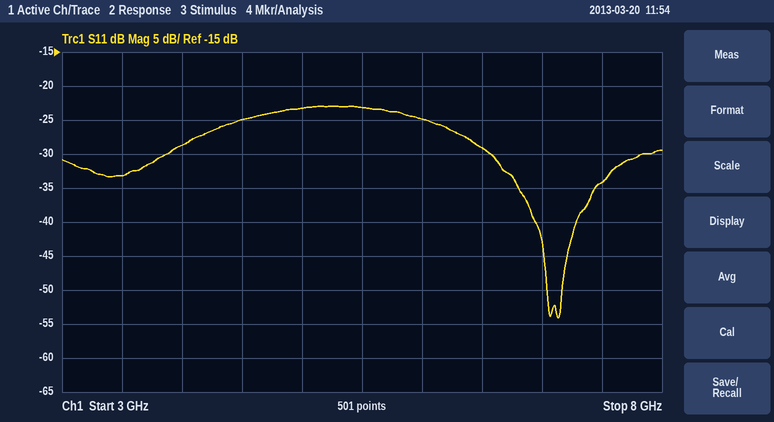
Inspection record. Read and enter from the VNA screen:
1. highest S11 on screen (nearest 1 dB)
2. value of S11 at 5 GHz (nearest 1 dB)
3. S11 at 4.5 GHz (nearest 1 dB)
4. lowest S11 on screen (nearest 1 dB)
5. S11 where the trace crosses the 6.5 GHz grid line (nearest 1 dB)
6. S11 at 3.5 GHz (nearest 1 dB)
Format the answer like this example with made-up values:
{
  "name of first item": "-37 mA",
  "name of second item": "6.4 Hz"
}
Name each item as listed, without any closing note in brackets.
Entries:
{
  "highest S11 on screen": "-23 dB",
  "value of S11 at 5 GHz": "-23 dB",
  "S11 at 4.5 GHz": "-25 dB",
  "lowest S11 on screen": "-54 dB",
  "S11 where the trace crosses the 6.5 GHz grid line": "-29 dB",
  "S11 at 3.5 GHz": "-33 dB"
}
